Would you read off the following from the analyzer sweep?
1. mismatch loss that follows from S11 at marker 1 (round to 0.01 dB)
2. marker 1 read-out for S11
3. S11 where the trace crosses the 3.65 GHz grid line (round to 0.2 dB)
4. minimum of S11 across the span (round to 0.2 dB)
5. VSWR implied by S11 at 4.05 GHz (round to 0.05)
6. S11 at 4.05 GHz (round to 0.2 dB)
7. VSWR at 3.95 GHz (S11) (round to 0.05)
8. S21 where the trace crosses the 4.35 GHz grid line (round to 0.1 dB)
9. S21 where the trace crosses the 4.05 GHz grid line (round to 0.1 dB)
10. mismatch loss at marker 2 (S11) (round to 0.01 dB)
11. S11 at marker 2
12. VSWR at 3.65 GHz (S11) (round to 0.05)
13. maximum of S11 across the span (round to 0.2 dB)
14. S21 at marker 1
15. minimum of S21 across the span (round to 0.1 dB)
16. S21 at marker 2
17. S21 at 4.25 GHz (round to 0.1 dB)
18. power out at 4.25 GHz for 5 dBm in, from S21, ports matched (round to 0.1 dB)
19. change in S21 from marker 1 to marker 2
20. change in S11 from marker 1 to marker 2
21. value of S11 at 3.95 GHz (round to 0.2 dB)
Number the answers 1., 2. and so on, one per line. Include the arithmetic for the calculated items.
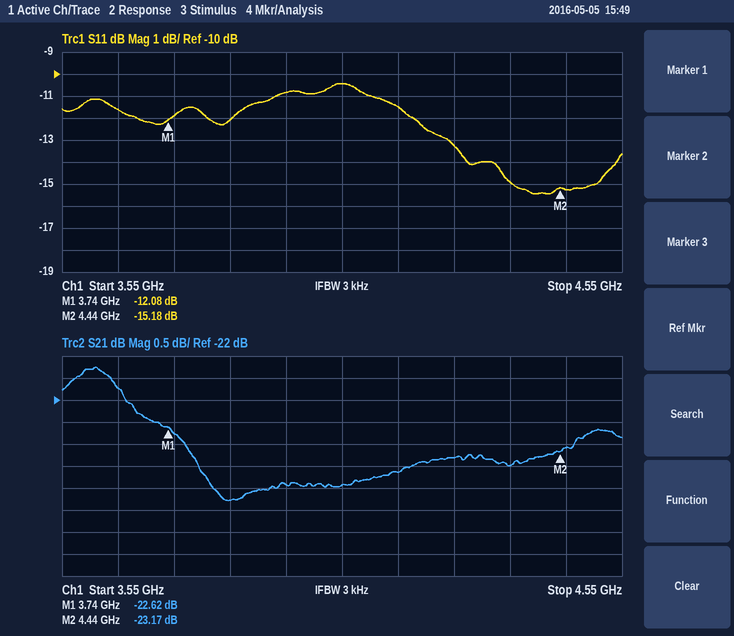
1. −10 log10(1 − 10^(-12.08/10)) ≈ 0.28 dB
2. -12.08 dB
3. -11.6 dB
4. -15.4 dB
5. |Γ| = 10^(-10.4/20) = 0.3020; VSWR = (1 + 0.3020)/(1 − 0.3020) ≈ 1.87, so 1.85 to the nearest 0.05
6. -10.4 dB
7. |Γ| = 10^(-10.8/20) = 0.2884; VSWR = (1 + 0.2884)/(1 − 0.2884) ≈ 1.81, so 1.80 to the nearest 0.05
8. -23.5 dB
9. -23.9 dB
10. −10 log10(1 − 10^(-15.18/10)) ≈ 0.13 dB
11. -15.18 dB
12. |Γ| = 10^(-11.6/20) = 0.2630; VSWR = (1 + 0.2630)/(1 − 0.2630) ≈ 1.71, so 1.70 to the nearest 0.05
13. -10.4 dB
14. -22.62 dB
15. -24.3 dB
16. -23.17 dB
17. -23.3 dB
18. 5 dBm + (-23.3 dB) = -18.3 dBm
19. -23.17 − (-22.62) = -0.55 dB
20. -15.18 − (-12.08) = -3.10 dB
21. -10.8 dB
